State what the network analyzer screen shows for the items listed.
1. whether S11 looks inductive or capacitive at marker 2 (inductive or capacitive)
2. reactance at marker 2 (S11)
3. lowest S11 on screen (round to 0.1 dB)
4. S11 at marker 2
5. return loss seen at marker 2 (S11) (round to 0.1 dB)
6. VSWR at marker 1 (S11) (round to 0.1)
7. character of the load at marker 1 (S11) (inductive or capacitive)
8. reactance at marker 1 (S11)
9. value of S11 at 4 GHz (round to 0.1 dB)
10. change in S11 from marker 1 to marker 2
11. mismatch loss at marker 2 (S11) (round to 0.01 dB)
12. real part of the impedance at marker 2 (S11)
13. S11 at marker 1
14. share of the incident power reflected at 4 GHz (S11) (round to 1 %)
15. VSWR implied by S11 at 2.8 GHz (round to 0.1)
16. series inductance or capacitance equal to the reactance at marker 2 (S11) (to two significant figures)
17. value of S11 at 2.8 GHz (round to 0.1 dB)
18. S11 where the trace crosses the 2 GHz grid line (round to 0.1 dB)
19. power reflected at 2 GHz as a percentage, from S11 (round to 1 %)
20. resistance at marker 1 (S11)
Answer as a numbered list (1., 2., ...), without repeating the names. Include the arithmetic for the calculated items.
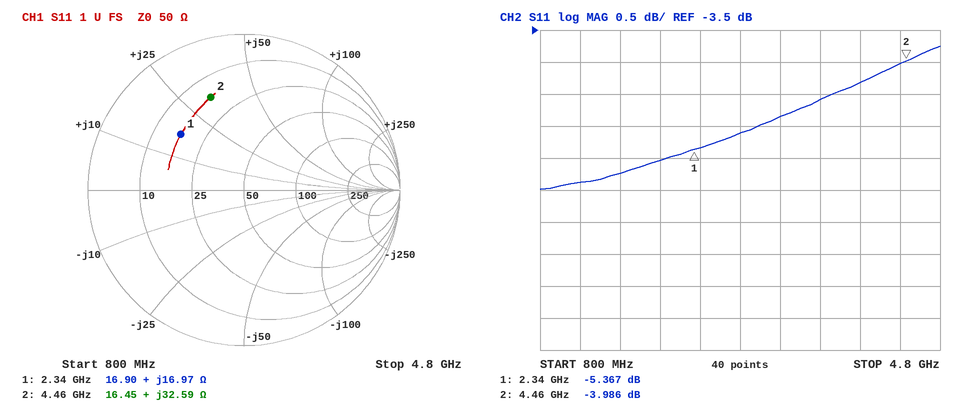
1. inductive
2. +32.59 Ω
3. -6.0 dB
4. -3.986 dB
5. 4.0 dB
6. 3.3
7. inductive
8. +16.97 Ω
9. -4.3 dB
10. -3.986 − (-5.367) = 1.381 dB
11. −10 log10(1 − 10^(-3.986/10)) ≈ 2.21 dB
12. 16.45 Ω
13. -5.367 dB
14. 10^(-4.3/10) ≈ 37 %
15. |Γ| = 10^(-5.1/20) = 0.5559; VSWR = (1 + 0.5559)/(1 − 0.5559) ≈ 3.5
16. L = 32.59 Ω/(2π × 4.46 GHz) ≈ 1.2 nH
17. -5.1 dB
18. -5.5 dB
19. 10^(-5.5/10) ≈ 28 %
20. 16.90 Ω
